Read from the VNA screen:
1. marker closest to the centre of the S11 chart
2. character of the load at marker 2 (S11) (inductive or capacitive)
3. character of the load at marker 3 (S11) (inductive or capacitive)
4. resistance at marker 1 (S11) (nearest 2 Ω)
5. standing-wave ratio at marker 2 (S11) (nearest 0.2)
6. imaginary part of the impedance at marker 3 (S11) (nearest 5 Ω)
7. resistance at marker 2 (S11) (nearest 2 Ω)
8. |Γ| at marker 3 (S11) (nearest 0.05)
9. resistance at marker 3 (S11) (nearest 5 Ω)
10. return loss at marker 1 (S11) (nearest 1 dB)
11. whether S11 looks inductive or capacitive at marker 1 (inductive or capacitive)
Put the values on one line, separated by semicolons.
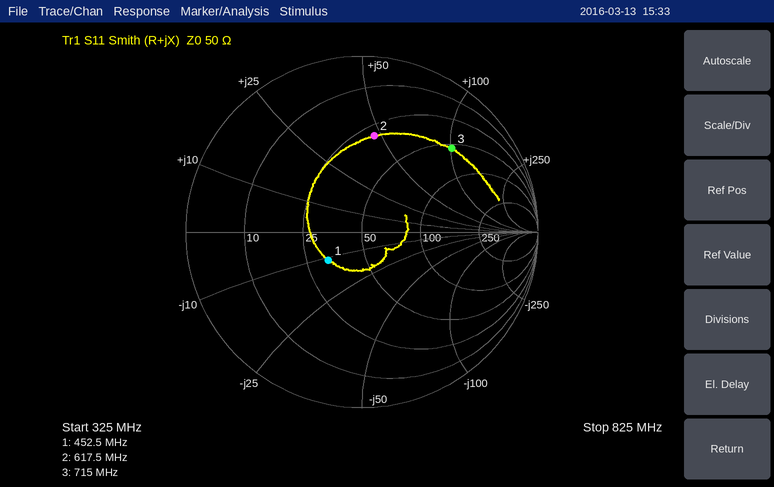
marker 1; inductive; inductive; 32 Ω; 3.4; +100 Ω; 30 Ω; 0.70; 55 Ω; 12 dB; capacitive
